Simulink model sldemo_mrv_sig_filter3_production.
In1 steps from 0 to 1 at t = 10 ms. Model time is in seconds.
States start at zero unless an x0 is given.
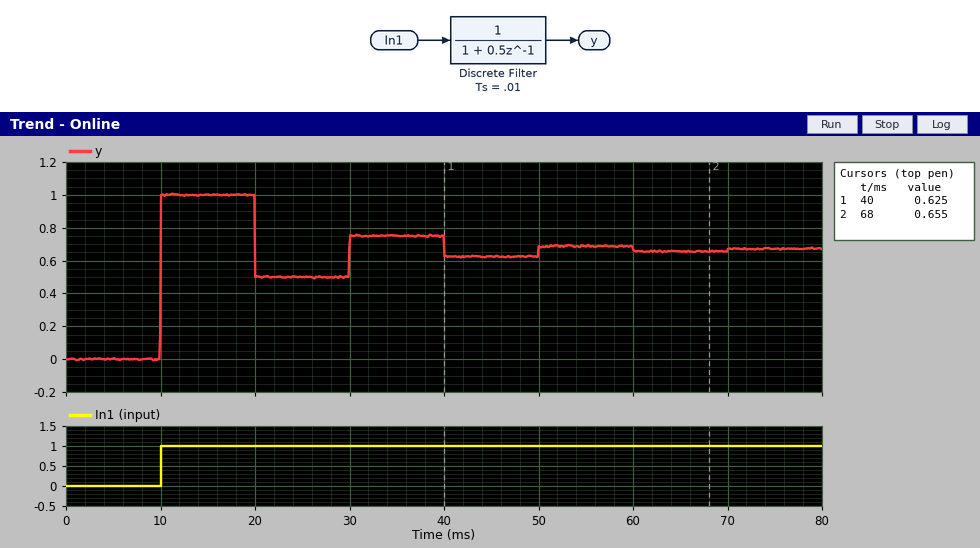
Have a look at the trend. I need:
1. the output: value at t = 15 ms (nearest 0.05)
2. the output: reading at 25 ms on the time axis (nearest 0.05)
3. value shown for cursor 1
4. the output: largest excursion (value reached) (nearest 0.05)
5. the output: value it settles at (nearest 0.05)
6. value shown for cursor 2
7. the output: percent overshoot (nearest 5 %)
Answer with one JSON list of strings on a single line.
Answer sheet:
["1.00", "0.50", "0.625", "1.00", "0.65", "0.655", "50 %"]
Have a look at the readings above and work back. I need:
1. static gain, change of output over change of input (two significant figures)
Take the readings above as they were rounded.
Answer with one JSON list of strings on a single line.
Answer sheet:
["0.65"]
